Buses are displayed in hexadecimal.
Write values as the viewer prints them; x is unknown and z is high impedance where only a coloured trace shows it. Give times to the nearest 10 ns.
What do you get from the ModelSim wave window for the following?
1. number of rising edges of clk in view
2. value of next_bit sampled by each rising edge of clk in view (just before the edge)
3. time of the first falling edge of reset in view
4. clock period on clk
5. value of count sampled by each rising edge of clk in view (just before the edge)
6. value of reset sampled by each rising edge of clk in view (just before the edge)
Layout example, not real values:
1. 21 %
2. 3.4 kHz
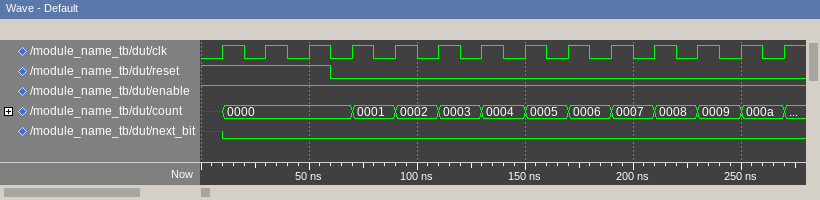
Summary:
1. 14
2. x 0 0 0 0 0 0 0 0 0 0 0 0 0
3. 60 ns
4. 20 ns
5. x, 0000, 0000, 0000, 0001, 0002, 0003, 0004, 0005, 0006, 0007, 0008, 0009, 000a
6. 1 1 1 0 0 0 0 0 0 0 0 0 0 0
